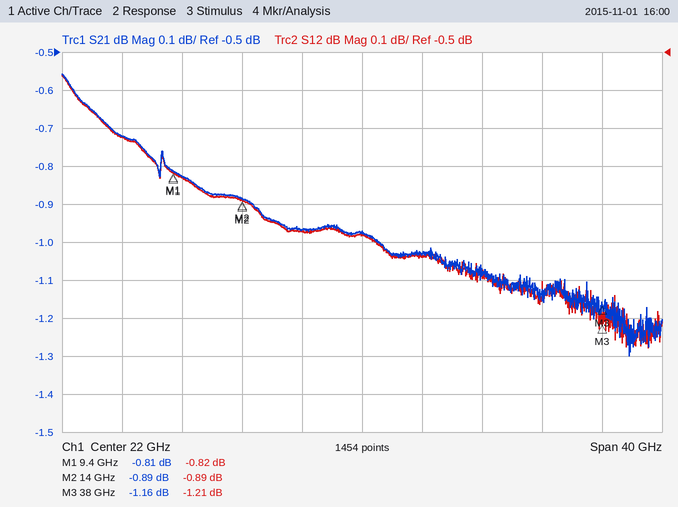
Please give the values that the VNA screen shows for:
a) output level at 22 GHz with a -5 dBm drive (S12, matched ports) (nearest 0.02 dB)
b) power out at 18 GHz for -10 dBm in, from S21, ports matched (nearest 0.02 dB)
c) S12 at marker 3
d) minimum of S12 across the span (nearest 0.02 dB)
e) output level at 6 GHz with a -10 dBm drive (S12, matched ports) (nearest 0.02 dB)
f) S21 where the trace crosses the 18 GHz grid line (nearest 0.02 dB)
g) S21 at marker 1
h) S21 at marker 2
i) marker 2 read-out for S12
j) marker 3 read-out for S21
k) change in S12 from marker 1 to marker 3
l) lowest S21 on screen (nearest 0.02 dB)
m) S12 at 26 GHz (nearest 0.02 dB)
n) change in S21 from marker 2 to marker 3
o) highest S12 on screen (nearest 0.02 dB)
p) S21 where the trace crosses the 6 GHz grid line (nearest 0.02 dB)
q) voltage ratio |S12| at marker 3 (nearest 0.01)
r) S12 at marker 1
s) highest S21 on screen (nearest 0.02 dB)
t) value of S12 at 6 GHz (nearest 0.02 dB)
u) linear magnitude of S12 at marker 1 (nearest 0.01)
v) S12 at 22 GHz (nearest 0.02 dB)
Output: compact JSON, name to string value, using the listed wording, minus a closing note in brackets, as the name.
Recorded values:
{"output level at 22 GHz with a -5 dBm drive (S12, matched ports)": "-5.98 dBm", "power out at 18 GHz for -10 dBm in, from S21, ports matched": "-10.96 dBm", "S12 at marker 3": "-1.21 dB", "minimum of S12 across the span": "-1.28 dB", "output level at 6 GHz with a -10 dBm drive (S12, matched ports)": "-10.72 dBm", "S21 where the trace crosses the 18 GHz grid line": "-0.96 dB", "S21 at marker 1": "-0.81 dB", "S21 at marker 2": "-0.89 dB", "marker 2 read-out for S12": "-0.89 dB", "marker 3 read-out for S21": "-1.16 dB", "change in S12 from marker 1 to marker 3": "-0.39 dB", "lowest S21 on screen": "-1.30 dB", "S12 at 26 GHz": "-1.04 dB", "change in S21 from marker 2 to marker 3": "-0.27 dB", "highest S12 on screen": "-0.56 dB", "S21 where the trace crosses the 6 GHz grid line": "-0.72 dB", "voltage ratio |S12| at marker 3": "0.87", "S12 at marker 1": "-0.82 dB", "highest S21 on screen": "-0.56 dB", "value of S12 at 6 GHz": "-0.72 dB", "linear magnitude of S12 at marker 1": "0.91", "S12 at 22 GHz": "-0.98 dB"}
